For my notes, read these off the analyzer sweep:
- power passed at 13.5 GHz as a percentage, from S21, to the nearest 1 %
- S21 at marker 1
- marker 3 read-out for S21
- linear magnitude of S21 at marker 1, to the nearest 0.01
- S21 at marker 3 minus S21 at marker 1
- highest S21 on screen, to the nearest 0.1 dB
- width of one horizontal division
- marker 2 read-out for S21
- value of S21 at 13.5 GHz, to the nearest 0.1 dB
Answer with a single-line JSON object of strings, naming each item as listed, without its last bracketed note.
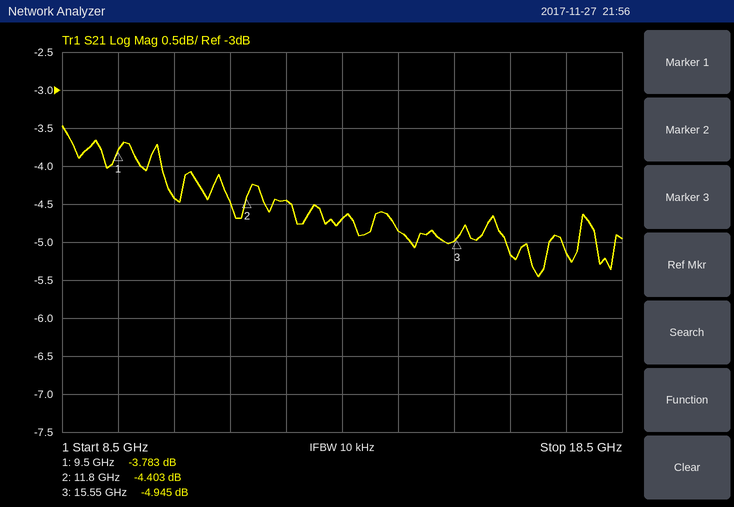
{"power passed at 13.5 GHz as a percentage, from S21, to the nearest 1 %": "34 %", "S21 at marker 1": "-3.783 dB", "marker 3 read-out for S21": "-4.945 dB", "linear magnitude of S21 at marker 1, to the nearest 0.01": "0.65", "S21 at marker 3 minus S21 at marker 1": "-1.162 dB", "highest S21 on screen, to the nearest 0.1 dB": "-3.5 dB", "width of one horizontal division": "1 GHz", "marker 2 read-out for S21": "-4.403 dB", "value of S21 at 13.5 GHz, to the nearest 0.1 dB": "-4.7 dB"}
